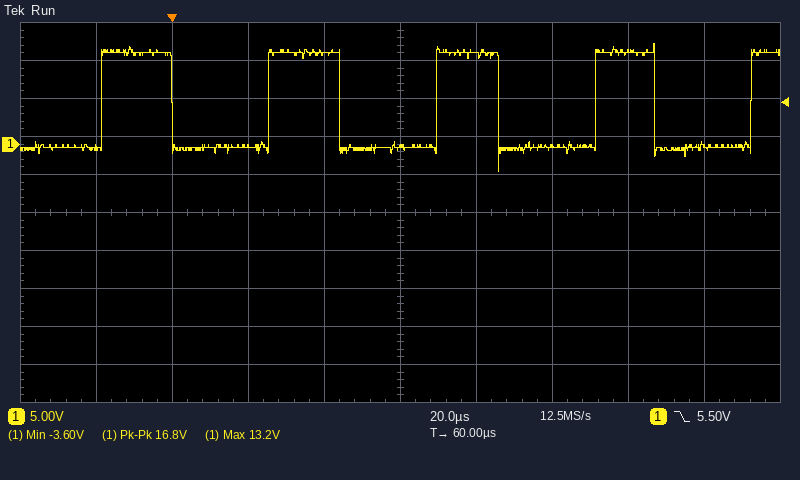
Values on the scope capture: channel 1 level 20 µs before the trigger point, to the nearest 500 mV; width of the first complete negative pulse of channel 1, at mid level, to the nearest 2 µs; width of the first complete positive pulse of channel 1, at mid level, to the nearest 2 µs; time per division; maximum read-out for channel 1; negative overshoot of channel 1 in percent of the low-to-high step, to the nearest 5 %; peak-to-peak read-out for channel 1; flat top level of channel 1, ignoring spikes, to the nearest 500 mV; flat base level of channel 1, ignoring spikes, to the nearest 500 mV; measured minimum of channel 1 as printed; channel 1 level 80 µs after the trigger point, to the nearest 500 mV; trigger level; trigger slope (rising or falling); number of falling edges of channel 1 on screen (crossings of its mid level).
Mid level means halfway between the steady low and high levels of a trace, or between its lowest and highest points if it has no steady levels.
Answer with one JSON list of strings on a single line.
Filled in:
["-500 mV", "26 µs", "18 µs", "20 µs", "13.2 V", "25 %", "16.8 V", "12.0 V", "-500 mV", "-3.60 V", "11.5 V", "5.50 V", "falling", "4"]
